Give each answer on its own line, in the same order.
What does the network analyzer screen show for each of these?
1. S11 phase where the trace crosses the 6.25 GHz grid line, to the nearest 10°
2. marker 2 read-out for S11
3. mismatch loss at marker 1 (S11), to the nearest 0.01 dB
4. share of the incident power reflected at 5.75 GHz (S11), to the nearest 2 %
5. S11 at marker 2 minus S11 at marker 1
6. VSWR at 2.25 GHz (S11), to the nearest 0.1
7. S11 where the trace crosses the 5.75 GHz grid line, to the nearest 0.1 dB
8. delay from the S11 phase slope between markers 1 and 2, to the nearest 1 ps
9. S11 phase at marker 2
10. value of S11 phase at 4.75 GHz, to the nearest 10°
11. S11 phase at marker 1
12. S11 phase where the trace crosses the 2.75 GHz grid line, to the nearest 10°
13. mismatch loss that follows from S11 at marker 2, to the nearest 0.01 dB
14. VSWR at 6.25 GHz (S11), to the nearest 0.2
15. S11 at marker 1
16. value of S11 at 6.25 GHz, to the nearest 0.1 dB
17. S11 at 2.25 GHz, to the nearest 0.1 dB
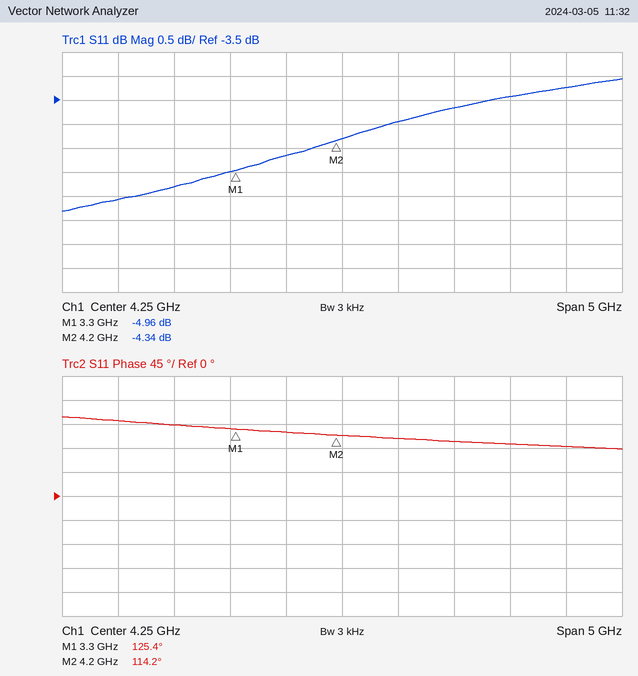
90°
-4.34 dB
1.67 dB
46 %
0.62 dB
3.2
-3.4 dB
35 ps
114.2°
110°
125.4°
130°
1.99 dB
5.4
-4.96 dB
-3.2 dB
-5.6 dB
